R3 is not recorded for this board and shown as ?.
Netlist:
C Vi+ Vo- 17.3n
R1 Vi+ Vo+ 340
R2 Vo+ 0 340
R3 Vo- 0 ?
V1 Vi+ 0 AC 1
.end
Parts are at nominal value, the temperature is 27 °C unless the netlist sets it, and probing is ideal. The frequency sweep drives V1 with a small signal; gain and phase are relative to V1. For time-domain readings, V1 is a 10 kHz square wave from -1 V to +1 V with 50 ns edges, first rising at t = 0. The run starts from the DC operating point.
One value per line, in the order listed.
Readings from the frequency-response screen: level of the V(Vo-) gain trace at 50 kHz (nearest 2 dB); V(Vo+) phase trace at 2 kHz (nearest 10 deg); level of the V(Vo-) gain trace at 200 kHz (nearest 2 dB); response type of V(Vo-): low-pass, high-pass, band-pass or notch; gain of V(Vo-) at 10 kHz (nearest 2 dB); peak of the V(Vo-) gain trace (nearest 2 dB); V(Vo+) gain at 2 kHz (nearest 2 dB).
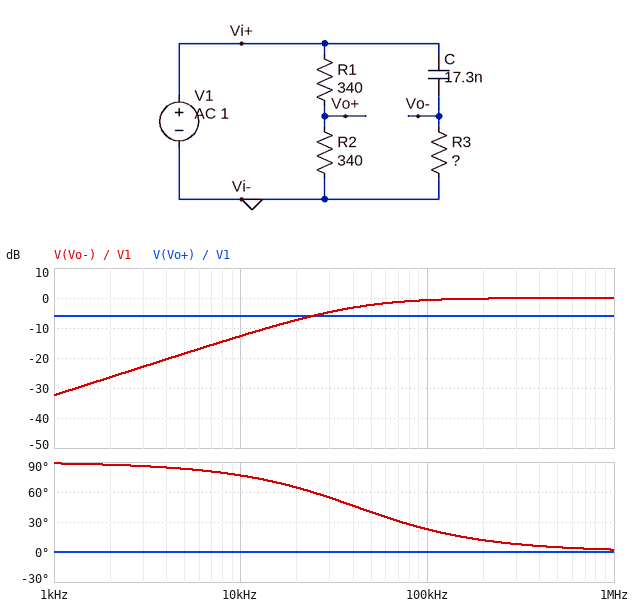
-2 dB
0 deg
0 dB
high-pass
-12 dB
0 dB
-6 dB
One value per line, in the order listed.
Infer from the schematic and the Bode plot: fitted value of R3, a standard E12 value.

220 Ω
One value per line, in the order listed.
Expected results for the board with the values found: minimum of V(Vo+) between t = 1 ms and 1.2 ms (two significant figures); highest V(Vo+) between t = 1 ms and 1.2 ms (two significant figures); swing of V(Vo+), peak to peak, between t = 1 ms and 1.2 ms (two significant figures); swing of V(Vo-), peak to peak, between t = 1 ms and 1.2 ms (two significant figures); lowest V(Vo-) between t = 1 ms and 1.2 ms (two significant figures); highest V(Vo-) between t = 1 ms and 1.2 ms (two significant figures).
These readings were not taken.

-500 mV
500 mV
1.0 V
4.0 V
-2.0 V
2.0 V
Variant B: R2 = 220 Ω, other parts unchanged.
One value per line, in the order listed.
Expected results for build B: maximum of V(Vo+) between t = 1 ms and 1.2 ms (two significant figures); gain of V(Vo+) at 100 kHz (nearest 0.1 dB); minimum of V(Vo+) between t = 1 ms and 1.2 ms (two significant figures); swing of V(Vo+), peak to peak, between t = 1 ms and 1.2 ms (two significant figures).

390 mV
-8.1 dB
-390 mV
790 mV
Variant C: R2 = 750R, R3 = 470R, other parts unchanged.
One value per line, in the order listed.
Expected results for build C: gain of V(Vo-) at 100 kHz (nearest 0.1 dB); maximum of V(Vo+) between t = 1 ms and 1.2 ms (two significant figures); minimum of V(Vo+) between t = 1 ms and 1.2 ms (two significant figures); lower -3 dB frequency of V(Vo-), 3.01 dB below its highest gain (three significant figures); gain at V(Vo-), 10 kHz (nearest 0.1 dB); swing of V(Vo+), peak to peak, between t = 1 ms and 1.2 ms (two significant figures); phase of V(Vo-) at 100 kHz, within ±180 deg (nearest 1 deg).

-0.2 dB
690 mV
-690 mV
19.6 kHz
-6.8 dB
1.4 V
11 deg
